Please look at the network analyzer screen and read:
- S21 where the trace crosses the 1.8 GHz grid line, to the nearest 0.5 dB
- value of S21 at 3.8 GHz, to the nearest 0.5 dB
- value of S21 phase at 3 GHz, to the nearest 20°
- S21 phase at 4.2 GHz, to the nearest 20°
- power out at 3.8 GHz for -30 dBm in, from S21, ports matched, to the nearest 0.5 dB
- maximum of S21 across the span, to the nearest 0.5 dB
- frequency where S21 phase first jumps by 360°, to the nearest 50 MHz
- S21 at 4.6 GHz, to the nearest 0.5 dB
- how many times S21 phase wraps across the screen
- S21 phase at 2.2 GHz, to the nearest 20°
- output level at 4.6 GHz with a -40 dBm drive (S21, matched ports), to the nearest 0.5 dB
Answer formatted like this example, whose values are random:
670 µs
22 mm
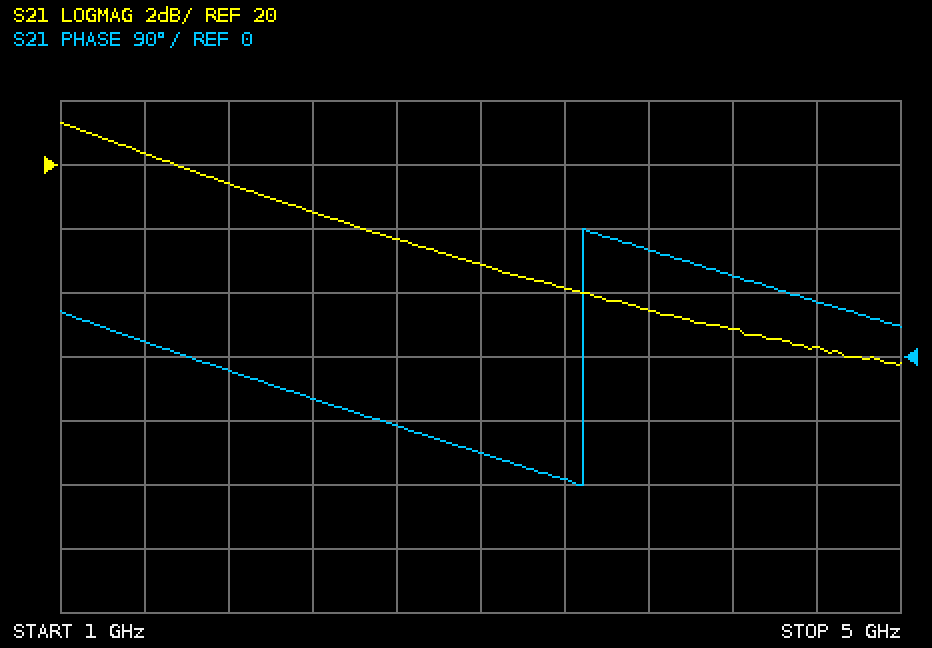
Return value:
19.5 dB
15.5 dB
-140°
120°
-14.5 dBm
21.5 dB
3.50 GHz
14.5 dB
1
-60°
-25.5 dBm
